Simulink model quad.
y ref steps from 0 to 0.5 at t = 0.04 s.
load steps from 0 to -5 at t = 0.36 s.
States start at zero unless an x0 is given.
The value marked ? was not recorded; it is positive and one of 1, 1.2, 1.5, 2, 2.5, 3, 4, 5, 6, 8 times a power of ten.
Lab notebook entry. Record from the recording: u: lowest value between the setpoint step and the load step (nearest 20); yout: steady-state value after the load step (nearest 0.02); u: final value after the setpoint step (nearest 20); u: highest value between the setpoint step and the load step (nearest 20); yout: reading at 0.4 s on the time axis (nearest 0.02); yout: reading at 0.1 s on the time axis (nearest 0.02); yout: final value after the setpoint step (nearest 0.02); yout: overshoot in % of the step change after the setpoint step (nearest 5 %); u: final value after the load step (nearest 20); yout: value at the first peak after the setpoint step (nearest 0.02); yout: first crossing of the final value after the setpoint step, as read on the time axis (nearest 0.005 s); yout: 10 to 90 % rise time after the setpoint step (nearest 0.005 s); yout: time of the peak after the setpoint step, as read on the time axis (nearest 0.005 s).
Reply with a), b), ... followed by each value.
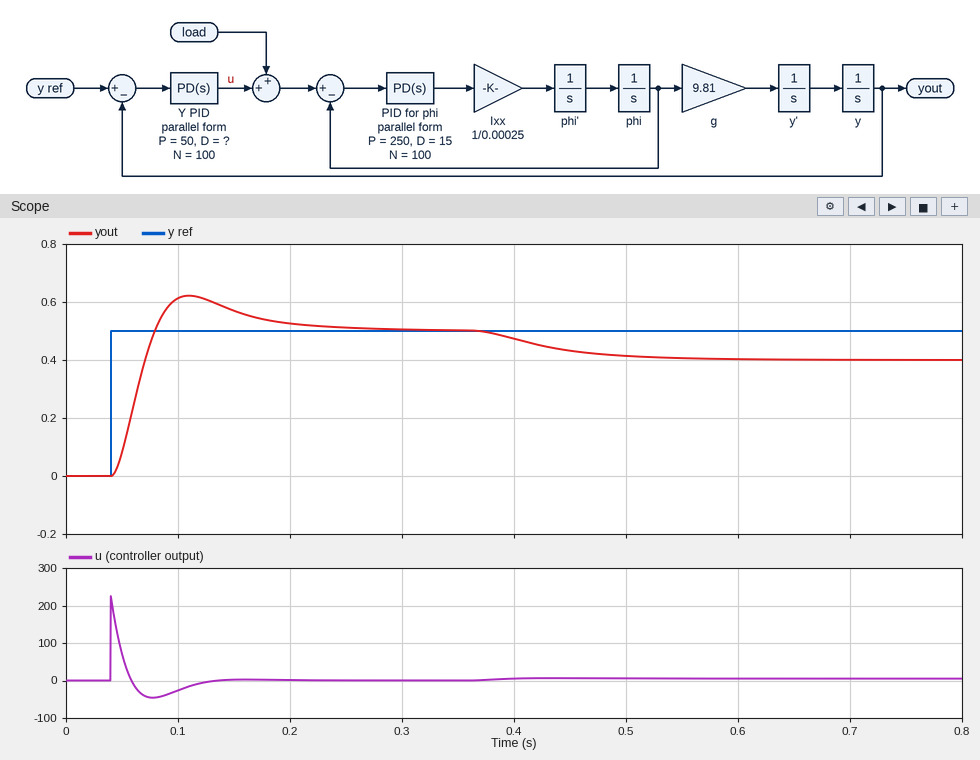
a) -40
b) 0.40
c) 0
d) 220
e) 0.48
f) 0.62
g) 0.50
h) 25 %
i) 0
j) 0.62
k) 0.080 s
l) 0.025 s
m) 0.110 s
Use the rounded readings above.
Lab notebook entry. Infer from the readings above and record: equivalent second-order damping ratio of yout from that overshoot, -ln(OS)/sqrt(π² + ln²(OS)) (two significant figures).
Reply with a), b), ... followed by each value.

a) 0.40
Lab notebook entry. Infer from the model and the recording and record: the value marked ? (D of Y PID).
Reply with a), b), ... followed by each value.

a) 4
